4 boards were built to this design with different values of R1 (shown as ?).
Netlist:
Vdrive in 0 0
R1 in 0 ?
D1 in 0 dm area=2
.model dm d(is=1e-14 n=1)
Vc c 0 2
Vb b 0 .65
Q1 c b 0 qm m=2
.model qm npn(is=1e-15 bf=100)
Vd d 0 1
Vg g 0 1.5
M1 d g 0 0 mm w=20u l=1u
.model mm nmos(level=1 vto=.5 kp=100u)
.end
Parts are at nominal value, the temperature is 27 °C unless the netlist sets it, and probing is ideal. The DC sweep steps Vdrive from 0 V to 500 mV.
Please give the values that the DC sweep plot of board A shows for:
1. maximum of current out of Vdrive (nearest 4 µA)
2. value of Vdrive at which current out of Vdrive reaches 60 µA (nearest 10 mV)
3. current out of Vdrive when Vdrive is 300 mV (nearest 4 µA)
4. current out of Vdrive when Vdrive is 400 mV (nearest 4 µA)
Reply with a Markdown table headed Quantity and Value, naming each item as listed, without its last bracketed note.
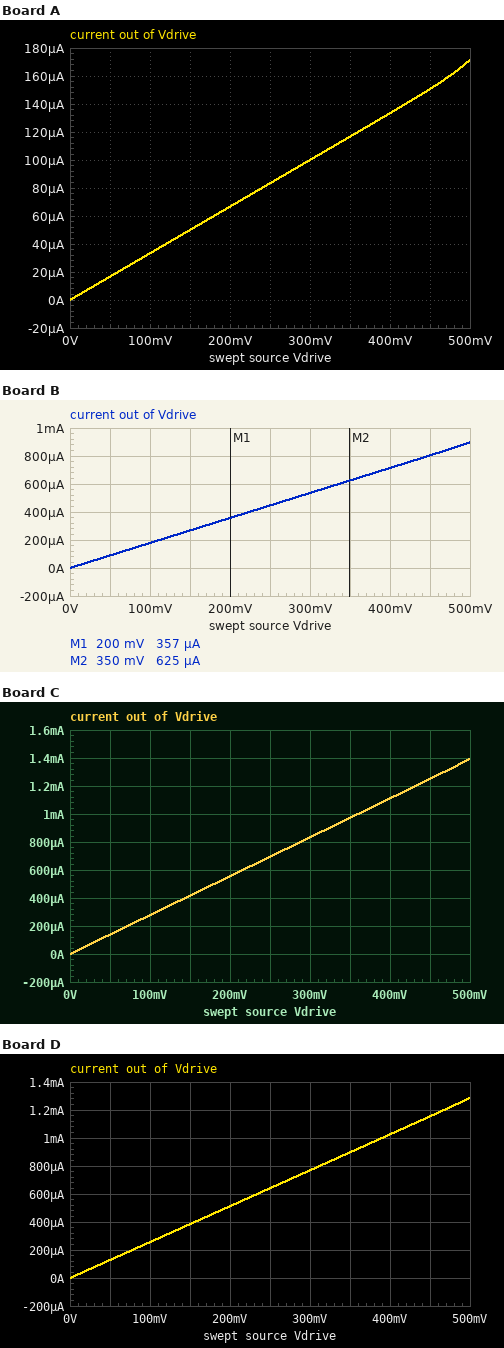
| Quantity | Value |
|---|---|
| maximum of current out of Vdrive | 172 µA |
| value of Vdrive at which current out of Vdrive reaches 60 µA | 180 mV |
| current out of Vdrive when Vdrive is 300 mV | 100 µA |
| current out of Vdrive when Vdrive is 400 mV | 132 µA |
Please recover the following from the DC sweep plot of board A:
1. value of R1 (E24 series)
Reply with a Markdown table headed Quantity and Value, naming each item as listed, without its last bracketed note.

| Quantity | Value |
|---|---|
| value of R1 | 3 kΩ |
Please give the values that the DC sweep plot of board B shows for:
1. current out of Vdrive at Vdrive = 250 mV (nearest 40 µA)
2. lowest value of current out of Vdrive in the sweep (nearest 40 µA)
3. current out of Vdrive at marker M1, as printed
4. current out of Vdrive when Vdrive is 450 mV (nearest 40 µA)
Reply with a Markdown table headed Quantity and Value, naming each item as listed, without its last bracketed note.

| Quantity | Value |
|---|---|
| current out of Vdrive at Vdrive = 250 mV | 440 µA |
| lowest value of current out of Vdrive in the sweep | 0 A |
| current out of Vdrive at marker M1, as printed | 357 µA |
| current out of Vdrive when Vdrive is 450 mV | 800 µA |
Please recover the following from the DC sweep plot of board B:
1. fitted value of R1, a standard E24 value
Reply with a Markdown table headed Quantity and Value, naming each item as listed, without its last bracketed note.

| Quantity | Value |
|---|---|
| fitted value of R1, a standard E24 value | 560 Ω |
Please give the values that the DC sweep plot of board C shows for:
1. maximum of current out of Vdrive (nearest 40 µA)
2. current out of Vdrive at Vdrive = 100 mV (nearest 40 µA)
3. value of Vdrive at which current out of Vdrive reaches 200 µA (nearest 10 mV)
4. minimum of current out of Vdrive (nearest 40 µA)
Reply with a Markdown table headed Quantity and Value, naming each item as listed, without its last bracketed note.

| Quantity | Value |
|---|---|
| maximum of current out of Vdrive | 1.40 mA |
| current out of Vdrive at Vdrive = 100 mV | 280 µA |
| value of Vdrive at which current out of Vdrive reaches 200 µA | 70 mV |
| minimum of current out of Vdrive | 0 A |
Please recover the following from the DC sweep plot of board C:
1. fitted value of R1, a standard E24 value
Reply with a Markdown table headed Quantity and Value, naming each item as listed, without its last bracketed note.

| Quantity | Value |
|---|---|
| fitted value of R1, a standard E24 value | 360 Ω |
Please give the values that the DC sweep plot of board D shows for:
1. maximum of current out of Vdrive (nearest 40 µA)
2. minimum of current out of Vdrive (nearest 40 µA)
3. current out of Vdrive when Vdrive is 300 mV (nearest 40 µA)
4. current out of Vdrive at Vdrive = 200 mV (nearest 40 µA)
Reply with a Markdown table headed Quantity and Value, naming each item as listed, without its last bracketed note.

| Quantity | Value |
|---|---|
| maximum of current out of Vdrive | 1.28 mA |
| minimum of current out of Vdrive | 0 A |
| current out of Vdrive when Vdrive is 300 mV | 760 µA |
| current out of Vdrive at Vdrive = 200 mV | 520 µA |
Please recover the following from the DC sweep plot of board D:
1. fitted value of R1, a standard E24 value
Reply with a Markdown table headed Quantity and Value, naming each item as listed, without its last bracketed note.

| Quantity | Value |
|---|---|
| fitted value of R1, a standard E24 value | 390 Ω |
